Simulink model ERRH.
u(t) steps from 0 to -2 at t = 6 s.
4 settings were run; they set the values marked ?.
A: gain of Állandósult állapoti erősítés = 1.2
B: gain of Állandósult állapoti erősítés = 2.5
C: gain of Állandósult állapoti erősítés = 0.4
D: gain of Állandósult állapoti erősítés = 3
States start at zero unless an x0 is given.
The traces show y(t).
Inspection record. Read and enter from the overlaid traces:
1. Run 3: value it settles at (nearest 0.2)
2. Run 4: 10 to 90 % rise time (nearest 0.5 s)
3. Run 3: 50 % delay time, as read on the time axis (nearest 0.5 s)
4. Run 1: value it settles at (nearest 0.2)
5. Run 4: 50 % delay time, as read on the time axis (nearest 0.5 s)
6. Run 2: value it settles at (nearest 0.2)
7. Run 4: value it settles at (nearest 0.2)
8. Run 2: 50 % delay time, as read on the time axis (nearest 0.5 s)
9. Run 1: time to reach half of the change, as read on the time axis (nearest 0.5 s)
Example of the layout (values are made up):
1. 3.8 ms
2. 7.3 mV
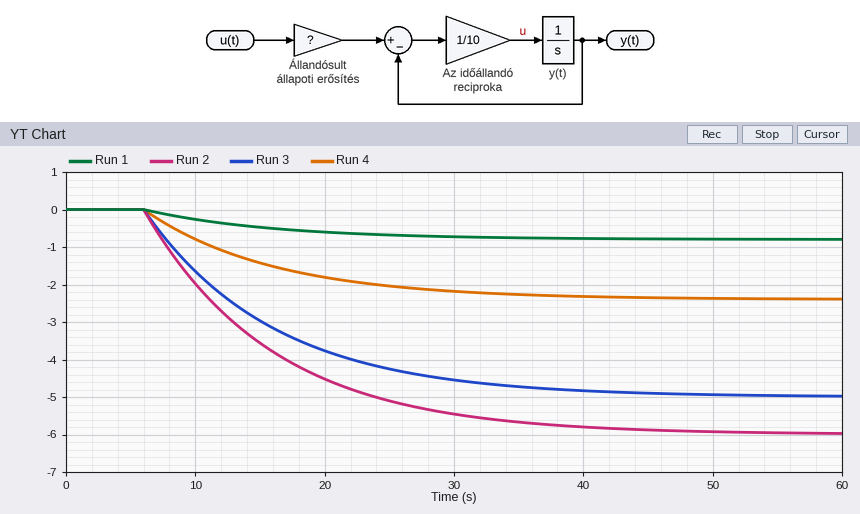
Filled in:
1. -5.0
2. 22.0 s
3. 13.0 s
4. -0.8
5. 13.0 s
6. -6.0
7. -2.4
8. 13.0 s
9. 13.0 s
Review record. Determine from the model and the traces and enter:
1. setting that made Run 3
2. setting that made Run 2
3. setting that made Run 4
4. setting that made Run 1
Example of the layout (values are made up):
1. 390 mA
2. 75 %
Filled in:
1. B
2. D
3. A
4. C
